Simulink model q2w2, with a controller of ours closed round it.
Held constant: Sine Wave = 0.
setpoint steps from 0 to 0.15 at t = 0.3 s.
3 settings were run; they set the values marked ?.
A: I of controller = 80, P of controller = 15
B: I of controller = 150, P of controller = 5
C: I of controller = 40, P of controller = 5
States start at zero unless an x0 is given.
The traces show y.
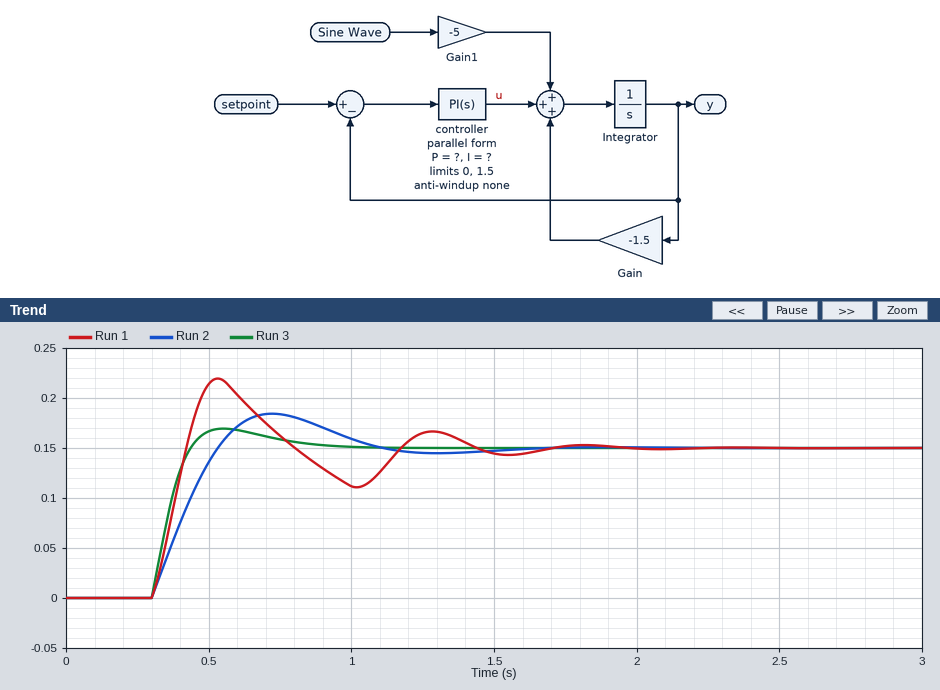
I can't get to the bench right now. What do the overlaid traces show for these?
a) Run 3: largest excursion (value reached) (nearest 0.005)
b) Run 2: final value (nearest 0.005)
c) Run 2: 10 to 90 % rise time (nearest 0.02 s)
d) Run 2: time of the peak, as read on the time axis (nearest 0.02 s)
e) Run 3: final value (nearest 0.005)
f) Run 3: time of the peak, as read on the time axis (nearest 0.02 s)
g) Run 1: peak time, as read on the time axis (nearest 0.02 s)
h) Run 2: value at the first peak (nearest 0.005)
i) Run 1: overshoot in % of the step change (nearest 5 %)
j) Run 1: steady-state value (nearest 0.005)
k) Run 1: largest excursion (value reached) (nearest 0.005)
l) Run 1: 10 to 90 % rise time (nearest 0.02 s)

0.170
0.150
0.18 s
0.72 s
0.150
0.56 s
0.54 s
0.185
45 %
0.150
0.220
0.10 s
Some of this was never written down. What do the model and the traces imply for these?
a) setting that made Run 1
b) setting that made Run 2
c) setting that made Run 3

B
C
A
